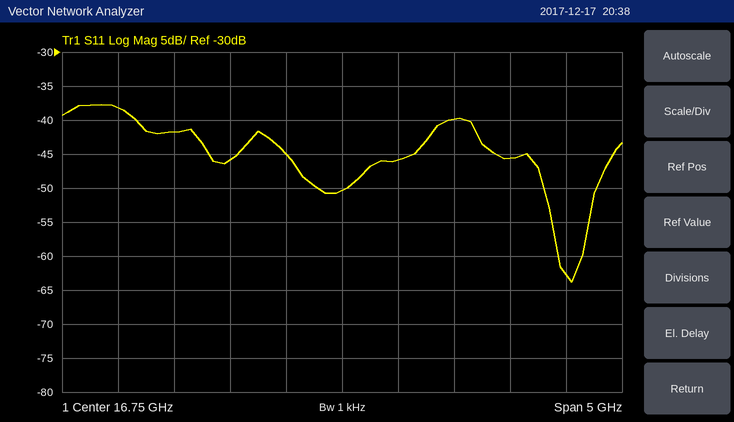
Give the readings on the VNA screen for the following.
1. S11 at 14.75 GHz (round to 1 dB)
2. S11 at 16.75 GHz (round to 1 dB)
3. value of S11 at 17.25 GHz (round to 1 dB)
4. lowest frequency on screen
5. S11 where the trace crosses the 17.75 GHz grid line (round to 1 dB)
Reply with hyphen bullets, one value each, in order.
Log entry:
- -38 dB
- -50 dB
- -46 dB
- 14.25 GHz
- -40 dB
